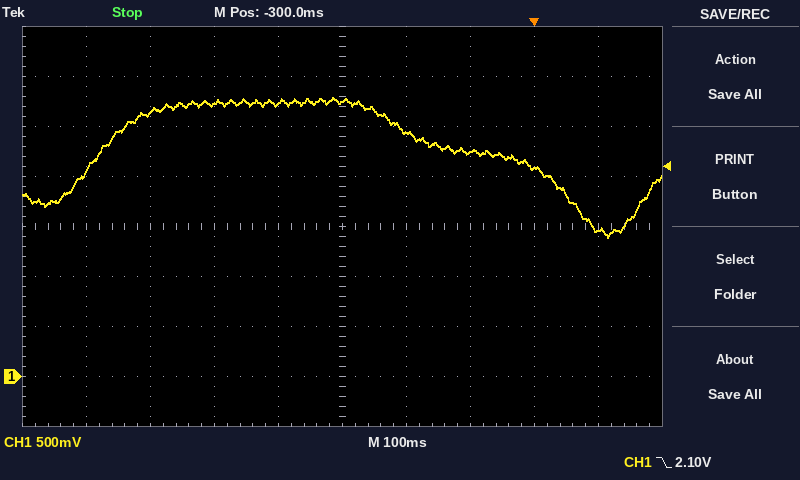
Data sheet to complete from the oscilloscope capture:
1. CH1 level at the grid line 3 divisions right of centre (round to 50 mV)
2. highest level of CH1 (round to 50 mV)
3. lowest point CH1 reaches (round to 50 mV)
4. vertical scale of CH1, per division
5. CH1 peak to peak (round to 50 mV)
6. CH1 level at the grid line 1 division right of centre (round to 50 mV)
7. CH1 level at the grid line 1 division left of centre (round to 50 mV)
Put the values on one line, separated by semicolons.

2.10 V; 2.80 V; 1.40 V; 500 mV; 1.40 V; 2.45 V; 2.75 V
